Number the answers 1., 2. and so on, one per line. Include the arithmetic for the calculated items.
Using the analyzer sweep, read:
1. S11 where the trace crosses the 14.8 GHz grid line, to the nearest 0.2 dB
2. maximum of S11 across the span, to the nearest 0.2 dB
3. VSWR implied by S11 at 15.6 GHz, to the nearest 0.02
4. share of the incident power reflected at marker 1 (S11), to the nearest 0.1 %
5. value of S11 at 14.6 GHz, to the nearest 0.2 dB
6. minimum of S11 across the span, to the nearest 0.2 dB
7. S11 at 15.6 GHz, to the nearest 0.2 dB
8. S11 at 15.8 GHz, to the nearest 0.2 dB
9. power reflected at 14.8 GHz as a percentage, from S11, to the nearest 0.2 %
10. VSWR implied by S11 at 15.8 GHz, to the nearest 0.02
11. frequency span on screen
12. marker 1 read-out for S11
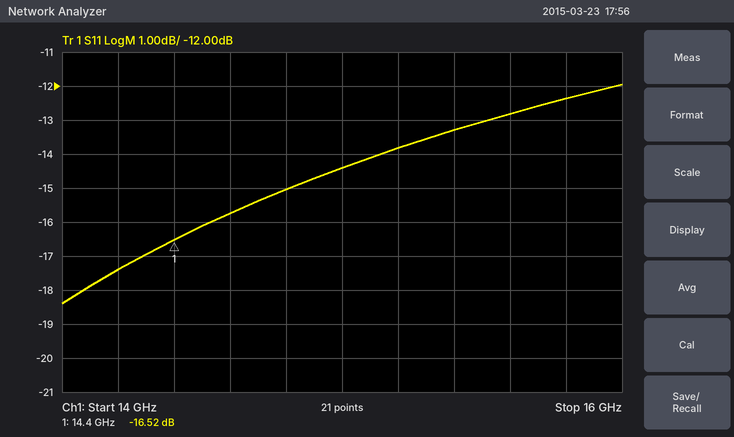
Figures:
1. -15.0 dB
2. -12.0 dB
3. |Γ| = 10^(-12.8/20) = 0.2291; VSWR = (1 + 0.2291)/(1 − 0.2291) ≈ 1.59, so 1.60 to the nearest 0.02
4. 10^(-16.52/10) ≈ 2.2 %
5. -15.8 dB
6. -18.4 dB
7. -12.8 dB
8. -12.4 dB
9. 10^(-15/10) ≈ 3.2 %
10. |Γ| = 10^(-12.4/20) = 0.2399; VSWR = (1 + 0.2399)/(1 − 0.2399) ≈ 1.63, so 1.64 to the nearest 0.02
11. 2 GHz
12. -16.52 dB
